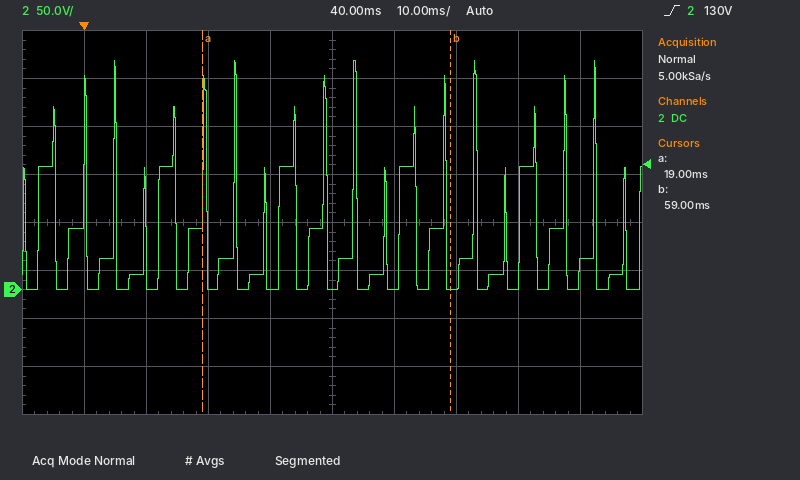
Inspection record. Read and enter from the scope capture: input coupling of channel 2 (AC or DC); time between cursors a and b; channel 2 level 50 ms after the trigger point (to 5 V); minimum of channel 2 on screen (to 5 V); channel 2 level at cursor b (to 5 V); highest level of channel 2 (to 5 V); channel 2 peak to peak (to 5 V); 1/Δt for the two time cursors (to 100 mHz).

DC
40 ms
0 V
0 V
0 V
240 V
240 V
25.0 Hz
